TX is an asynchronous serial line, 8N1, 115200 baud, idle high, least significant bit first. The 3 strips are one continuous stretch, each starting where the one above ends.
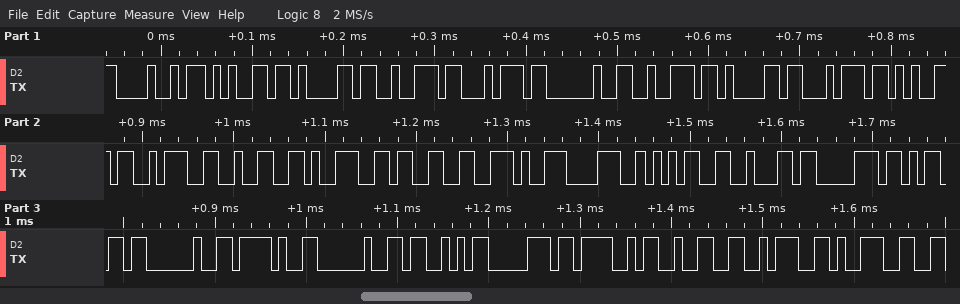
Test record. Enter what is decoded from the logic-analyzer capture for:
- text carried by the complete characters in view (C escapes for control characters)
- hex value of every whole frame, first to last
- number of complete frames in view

"Heart rate:293.85bpm / SpO2:9"
0x48 0x65 0x61 0x72 0x74 0x20 0x72 0x61 0x74 0x65 0x3A 0x32 0x39 0x33 0x2E 0x38 0x35 0x62 0x70 0x6D 0x20 0x2F 0x20 0x53 0x70 0x4F 0x32 0x3A 0x39
29
